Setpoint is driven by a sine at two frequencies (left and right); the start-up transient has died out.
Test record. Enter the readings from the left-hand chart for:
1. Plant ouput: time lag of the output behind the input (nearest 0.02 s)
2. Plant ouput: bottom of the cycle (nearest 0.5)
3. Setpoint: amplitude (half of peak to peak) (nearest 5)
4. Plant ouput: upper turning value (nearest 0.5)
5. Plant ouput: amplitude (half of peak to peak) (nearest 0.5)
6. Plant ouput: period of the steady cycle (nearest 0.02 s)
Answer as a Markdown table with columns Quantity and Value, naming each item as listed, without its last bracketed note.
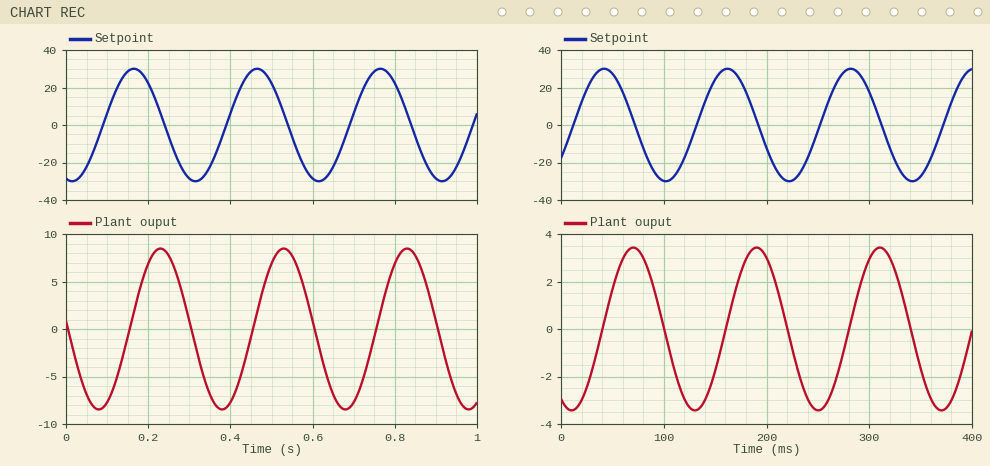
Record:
| Quantity | Value |
|---|---|
| Plant ouput: time lag of the output behind the input | 0.06 s |
| Plant ouput: bottom of the cycle | -8.5 |
| Setpoint: amplitude (half of peak to peak) | 30 |
| Plant ouput: upper turning value | 8.5 |
| Plant ouput: amplitude (half of peak to peak) | 8.5 |
| Plant ouput: period of the steady cycle | 0.30 s |
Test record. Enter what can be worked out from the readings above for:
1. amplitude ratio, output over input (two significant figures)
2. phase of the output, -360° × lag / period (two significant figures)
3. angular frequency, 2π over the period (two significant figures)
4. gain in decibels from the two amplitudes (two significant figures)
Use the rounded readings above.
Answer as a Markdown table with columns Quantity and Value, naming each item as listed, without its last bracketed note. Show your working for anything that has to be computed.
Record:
| Quantity | Value |
|---|---|
| amplitude ratio, output over input | 8.5 / 30 = 0.28 |
| phase of the output, -360° × lag / period | -360 × 0.06 / 0.3 = -72° |
| angular frequency, 2π over the period | 2π / 0.3 = 21 rad/s |
| gain in decibels from the two amplitudes | 20 log10(8.5 / 30) = -11 dB |
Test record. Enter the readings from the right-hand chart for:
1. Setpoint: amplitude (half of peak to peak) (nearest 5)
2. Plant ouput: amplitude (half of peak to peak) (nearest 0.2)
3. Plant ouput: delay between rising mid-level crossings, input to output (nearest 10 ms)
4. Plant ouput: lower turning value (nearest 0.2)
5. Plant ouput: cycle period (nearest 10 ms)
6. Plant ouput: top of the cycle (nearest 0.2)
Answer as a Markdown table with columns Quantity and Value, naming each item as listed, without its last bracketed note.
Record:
| Quantity | Value |
|---|---|
| Setpoint: amplitude (half of peak to peak) | 30 |
| Plant ouput: amplitude (half of peak to peak) | 3.4 |
| Plant ouput: delay between rising mid-level crossings, input to output | 30 ms |
| Plant ouput: lower turning value | -3.4 |
| Plant ouput: cycle period | 120 ms |
| Plant ouput: top of the cycle | 3.4 |
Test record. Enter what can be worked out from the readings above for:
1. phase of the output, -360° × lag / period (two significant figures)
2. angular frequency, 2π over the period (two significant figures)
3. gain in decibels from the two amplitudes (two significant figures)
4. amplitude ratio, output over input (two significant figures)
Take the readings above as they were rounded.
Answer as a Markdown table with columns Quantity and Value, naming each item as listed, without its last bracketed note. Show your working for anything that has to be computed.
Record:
| Quantity | Value |
|---|---|
| phase of the output, -360° × lag / period | -360 × 30 / 120 = -90° |
| angular frequency, 2π over the period | 2π / 120 = 0.052 rad/ms |
| gain in decibels from the two amplitudes | 20 log10(3.4 / 30) = -19 dB |
| amplitude ratio, output over input | 3.4 / 30 = 0.11 |
